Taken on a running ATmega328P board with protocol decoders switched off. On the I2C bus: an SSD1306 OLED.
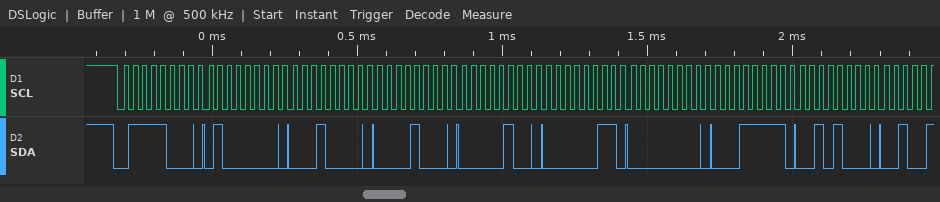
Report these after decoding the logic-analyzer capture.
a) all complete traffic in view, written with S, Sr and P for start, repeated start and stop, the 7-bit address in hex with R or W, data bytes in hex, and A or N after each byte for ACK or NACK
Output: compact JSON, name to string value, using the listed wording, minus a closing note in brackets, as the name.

{"all complete traffic in view, written with S, Sr and P for start, repeated start and stop, the 7-bit address in hex with R or W, data bytes in hex, and A or N after each byte for ACK or NACK": "S 3CW A 40 A 10 A 08 A 04 A 03 A 00 A 1F A 28 A"}
